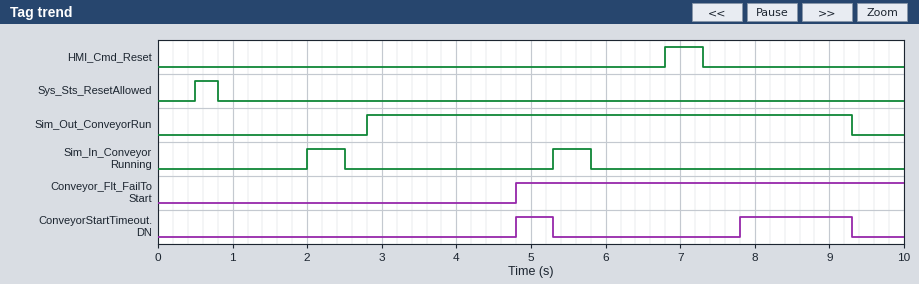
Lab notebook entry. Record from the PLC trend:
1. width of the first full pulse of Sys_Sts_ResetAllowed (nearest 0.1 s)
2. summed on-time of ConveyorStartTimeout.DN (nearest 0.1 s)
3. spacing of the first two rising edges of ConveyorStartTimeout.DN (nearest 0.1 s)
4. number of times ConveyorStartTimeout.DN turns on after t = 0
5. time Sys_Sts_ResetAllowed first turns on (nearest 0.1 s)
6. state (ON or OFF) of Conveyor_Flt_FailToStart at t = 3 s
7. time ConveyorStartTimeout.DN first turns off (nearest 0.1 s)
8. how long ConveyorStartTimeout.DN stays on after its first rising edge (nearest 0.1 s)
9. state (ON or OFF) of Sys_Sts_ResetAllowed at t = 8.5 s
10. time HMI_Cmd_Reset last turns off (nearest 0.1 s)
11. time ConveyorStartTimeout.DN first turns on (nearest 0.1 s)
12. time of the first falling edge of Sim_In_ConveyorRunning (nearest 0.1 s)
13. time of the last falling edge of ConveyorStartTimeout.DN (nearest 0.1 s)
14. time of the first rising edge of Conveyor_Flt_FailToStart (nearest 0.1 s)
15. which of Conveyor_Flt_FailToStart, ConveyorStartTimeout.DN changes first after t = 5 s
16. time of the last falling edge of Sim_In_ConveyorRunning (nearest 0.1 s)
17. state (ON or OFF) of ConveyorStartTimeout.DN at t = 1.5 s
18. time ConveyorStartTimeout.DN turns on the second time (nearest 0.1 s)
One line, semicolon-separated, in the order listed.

0.3 s; 2.0 s; 3.0 s; 2; 0.5 s; OFF; 5.3 s; 0.5 s; OFF; 7.3 s; 4.8 s; 2.5 s; 9.3 s; 4.8 s; ConveyorStartTimeout.DN; 5.8 s; OFF; 7.8 s
